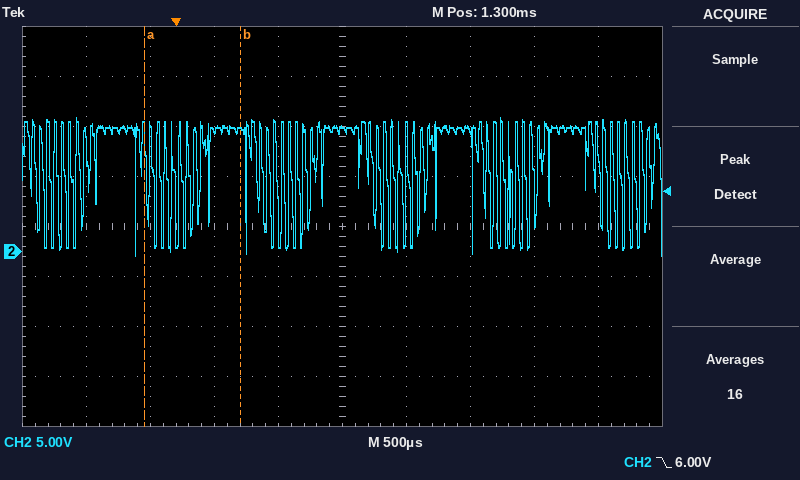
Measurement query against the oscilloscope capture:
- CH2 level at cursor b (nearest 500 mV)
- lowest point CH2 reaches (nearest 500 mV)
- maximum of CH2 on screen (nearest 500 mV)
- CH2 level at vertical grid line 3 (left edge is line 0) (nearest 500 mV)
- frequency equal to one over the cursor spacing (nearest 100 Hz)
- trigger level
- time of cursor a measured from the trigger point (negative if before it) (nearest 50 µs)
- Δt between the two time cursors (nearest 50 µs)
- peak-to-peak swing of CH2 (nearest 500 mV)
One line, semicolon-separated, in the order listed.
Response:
12.0 V; -500 mV; 13.5 V; 12.0 V; 1.3 kHz; 6.00 V; -250 µs; 750 µs; 14.0 V
